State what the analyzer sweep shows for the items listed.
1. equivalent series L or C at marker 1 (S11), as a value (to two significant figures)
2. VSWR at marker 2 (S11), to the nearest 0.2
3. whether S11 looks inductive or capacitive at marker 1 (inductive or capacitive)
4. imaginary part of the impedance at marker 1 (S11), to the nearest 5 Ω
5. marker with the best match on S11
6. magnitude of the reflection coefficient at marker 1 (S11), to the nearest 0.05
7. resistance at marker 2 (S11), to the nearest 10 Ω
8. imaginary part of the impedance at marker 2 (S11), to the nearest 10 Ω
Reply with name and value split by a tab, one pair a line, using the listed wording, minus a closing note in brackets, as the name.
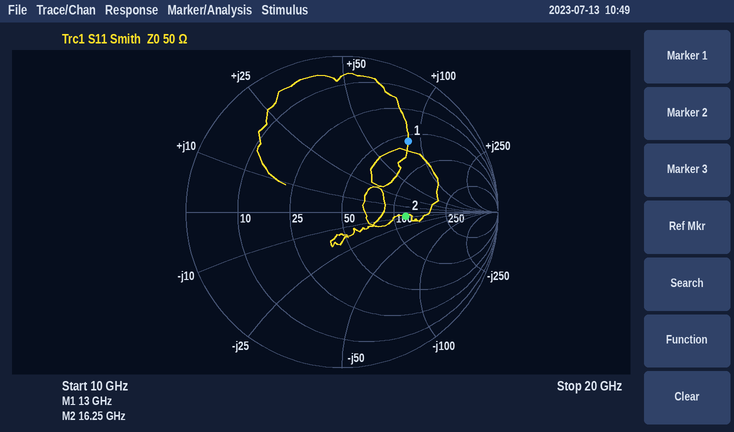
equivalent series L or C at marker 1 (S11), as a value	1.0 nH
VSWR at marker 2 (S11), to the nearest 0.2	2.4
whether S11 looks inductive or capacitive at marker 1	inductive
imaginary part of the impedance at marker 1 (S11), to the nearest 5 Ω	+85 Ω
marker with the best match on S11	marker 2
magnitude of the reflection coefficient at marker 1 (S11), to the nearest 0.05	0.60
resistance at marker 2 (S11), to the nearest 10 Ω	120 Ω
imaginary part of the impedance at marker 2 (S11), to the nearest 10 Ω	-10 Ω
